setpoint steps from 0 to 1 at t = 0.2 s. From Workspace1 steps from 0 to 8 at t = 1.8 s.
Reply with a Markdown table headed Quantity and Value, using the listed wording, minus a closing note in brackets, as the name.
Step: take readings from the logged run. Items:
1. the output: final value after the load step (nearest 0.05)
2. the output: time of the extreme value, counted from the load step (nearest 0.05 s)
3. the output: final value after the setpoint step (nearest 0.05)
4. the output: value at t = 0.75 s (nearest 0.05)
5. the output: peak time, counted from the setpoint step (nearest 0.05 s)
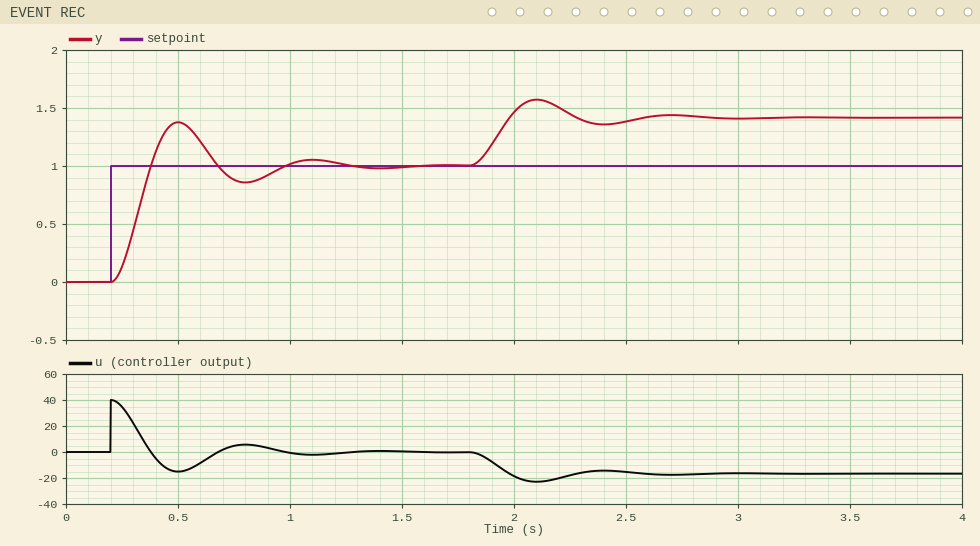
| Quantity | Value |
|---|---|
| the output: final value after the load step | 1.40 |
| the output: time of the extreme value, counted from the load step | 0.30 s |
| the output: final value after the setpoint step | 1.00 |
| the output: value at t = 0.75 s | 0.90 |
| the output: peak time, counted from the setpoint step | 0.30 s |
